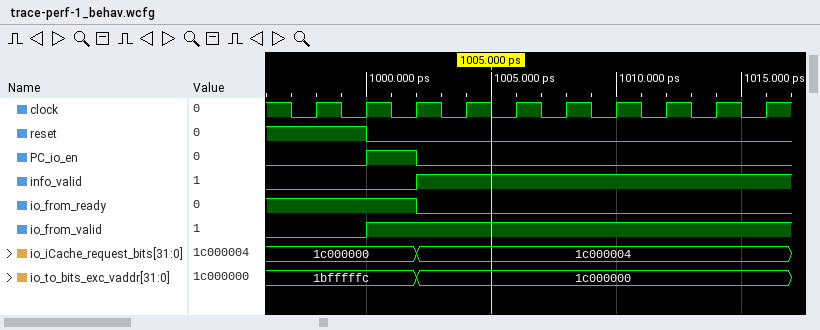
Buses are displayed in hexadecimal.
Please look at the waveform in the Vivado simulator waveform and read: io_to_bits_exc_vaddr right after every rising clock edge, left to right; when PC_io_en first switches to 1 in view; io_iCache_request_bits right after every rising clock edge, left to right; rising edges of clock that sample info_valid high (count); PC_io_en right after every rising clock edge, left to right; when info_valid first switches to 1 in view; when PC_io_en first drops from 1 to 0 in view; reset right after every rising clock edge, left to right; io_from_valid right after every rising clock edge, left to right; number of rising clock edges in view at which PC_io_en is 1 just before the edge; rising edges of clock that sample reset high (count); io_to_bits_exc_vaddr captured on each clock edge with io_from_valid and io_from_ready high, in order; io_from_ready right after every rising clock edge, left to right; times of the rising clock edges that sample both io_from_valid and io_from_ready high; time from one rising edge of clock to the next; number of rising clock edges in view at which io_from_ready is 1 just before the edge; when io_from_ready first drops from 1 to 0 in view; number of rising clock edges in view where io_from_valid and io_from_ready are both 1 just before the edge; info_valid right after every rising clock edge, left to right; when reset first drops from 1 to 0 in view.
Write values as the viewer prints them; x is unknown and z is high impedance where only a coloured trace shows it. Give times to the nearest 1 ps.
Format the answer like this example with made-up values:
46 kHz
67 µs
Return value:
1bfffffc, 1bfffffc, 1c000000, 1c000000, 1c000000, 1c000000, 1c000000, 1c000000, 1c000000, 1c000000
1000 ps
1c000000, 1c000000, 1c000004, 1c000004, 1c000004, 1c000004, 1c000004, 1c000004, 1c000004, 1c000004
7
0 1 0 0 0 0 0 0 0 0
1002 ps
1002 ps
1 0 0 0 0 0 0 0 0 0
0 1 1 1 1 1 1 1 1 1
1
2
1bfffffc
1 1 0 0 0 0 0 0 0 0
1002 ps
2 ps
3
1002 ps
1
0 0 1 1 1 1 1 1 1 1
1000 ps
